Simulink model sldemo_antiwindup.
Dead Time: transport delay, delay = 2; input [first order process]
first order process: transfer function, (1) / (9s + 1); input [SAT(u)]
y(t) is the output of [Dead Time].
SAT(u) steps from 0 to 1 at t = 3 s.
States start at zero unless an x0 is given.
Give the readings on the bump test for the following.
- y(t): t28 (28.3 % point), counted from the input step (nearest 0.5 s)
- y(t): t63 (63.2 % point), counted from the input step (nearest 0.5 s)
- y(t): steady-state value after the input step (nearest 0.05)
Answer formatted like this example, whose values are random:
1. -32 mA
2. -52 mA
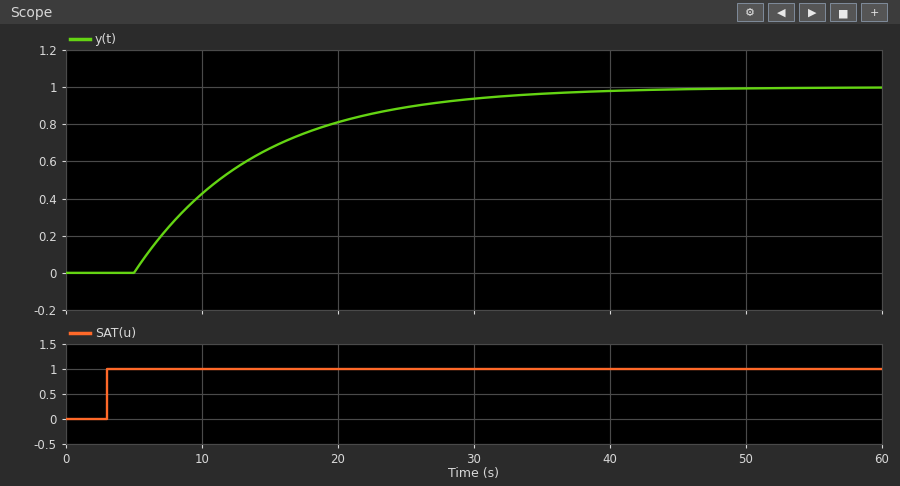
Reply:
1. 5.0 s
2. 11.0 s
3. 1.00
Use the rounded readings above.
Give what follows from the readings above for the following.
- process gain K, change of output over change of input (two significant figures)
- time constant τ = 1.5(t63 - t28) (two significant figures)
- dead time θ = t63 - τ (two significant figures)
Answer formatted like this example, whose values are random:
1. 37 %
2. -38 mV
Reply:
1. 1.0
2. 9.0 s
3. 2.0 s
